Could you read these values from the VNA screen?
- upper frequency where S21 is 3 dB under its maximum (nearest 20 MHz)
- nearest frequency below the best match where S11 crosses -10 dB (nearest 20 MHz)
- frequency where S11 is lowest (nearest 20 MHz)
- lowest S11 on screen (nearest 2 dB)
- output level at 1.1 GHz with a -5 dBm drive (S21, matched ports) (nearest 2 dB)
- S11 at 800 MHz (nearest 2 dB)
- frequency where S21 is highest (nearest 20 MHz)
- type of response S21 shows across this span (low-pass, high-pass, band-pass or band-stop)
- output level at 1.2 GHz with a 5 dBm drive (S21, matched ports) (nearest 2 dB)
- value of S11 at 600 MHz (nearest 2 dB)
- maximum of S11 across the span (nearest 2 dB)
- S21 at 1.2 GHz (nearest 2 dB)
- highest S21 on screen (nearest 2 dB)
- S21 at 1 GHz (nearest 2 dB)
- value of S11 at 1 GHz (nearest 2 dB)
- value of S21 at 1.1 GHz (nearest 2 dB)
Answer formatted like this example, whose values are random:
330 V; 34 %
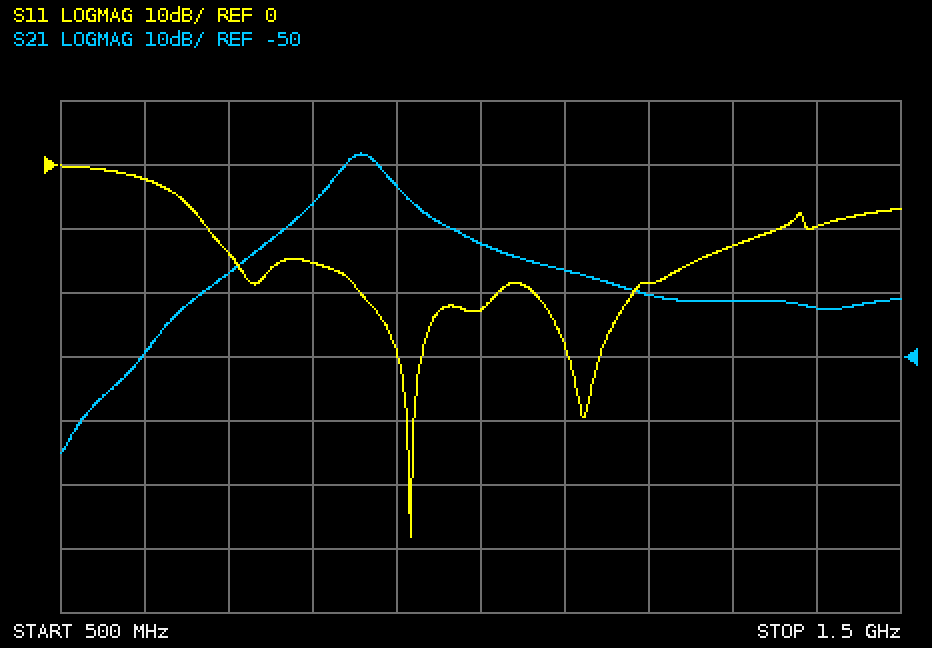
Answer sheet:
880 MHz; 680 MHz; 920 MHz; -58 dB; -42 dBm; -16 dB; 860 MHz; band-pass; -36 dBm; -2 dB; 0 dB; -40 dB; -18 dB; -32 dB; -22 dB; -36 dB
